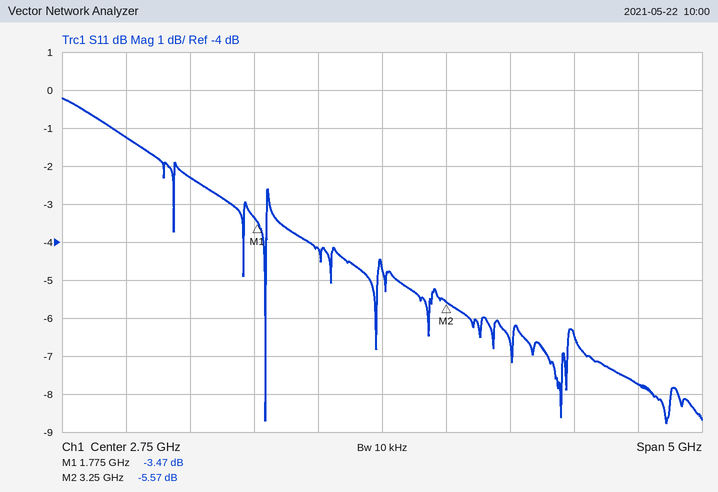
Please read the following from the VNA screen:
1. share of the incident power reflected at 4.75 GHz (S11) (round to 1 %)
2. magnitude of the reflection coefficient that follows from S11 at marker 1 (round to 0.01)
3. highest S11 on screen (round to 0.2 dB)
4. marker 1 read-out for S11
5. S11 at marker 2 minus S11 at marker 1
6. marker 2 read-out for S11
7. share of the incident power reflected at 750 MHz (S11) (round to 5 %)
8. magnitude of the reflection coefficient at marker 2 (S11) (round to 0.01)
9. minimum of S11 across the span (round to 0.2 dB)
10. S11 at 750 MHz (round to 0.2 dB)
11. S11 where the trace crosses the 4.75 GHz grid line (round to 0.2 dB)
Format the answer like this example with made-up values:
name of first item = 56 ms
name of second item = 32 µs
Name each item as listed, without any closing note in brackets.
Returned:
share of the incident power reflected at 4.75 GHz (S11) = 17 %
magnitude of the reflection coefficient that follows from S11 at marker 1 = 0.67
highest S11 on screen = -0.2 dB
marker 1 read-out for S11 = -3.47 dB
S11 at marker 2 minus S11 at marker 1 = -2.10 dB
marker 2 read-out for S11 = -5.57 dB
share of the incident power reflected at 750 MHz (S11) = 75 %
magnitude of the reflection coefficient at marker 2 (S11) = 0.53
minimum of S11 across the span = -8.8 dB
S11 at 750 MHz = -1.2 dB
S11 where the trace crosses the 4.75 GHz grid line = -7.8 dB
